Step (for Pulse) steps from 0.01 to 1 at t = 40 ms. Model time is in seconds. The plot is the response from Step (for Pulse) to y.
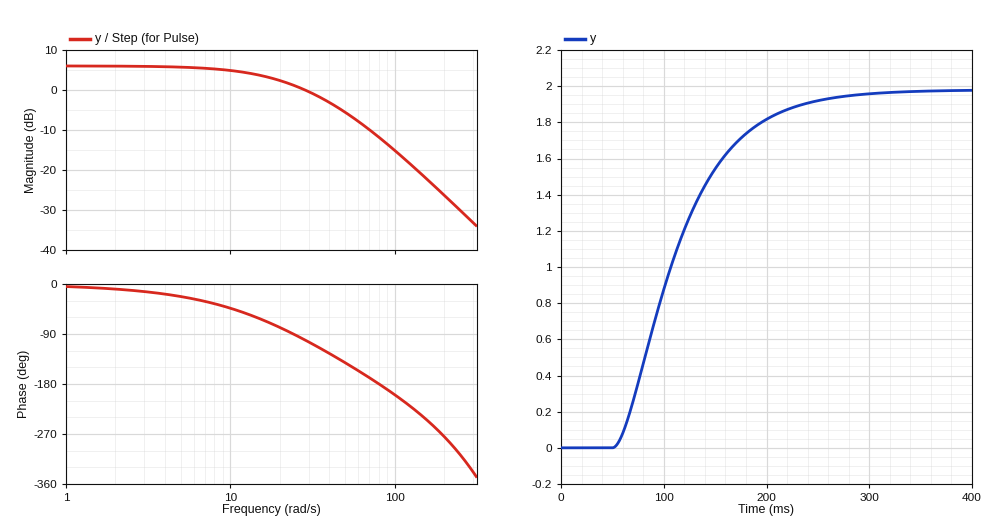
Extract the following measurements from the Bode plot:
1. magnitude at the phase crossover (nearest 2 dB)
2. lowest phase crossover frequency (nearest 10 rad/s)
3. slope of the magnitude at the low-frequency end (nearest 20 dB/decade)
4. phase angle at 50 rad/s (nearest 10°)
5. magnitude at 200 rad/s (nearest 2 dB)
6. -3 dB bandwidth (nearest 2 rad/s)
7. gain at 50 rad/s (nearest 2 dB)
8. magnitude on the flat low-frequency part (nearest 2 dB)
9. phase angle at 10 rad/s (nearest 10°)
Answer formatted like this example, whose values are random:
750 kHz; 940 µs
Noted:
-12 dB; 80 rad/s; 0 dB/decade; -140°; -26 dB; 18 rad/s; -6 dB; 6 dB; -40°
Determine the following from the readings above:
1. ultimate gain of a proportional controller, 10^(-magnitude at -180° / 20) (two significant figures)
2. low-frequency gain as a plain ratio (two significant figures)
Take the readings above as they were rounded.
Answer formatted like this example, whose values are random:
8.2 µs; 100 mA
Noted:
4.0; 2.0
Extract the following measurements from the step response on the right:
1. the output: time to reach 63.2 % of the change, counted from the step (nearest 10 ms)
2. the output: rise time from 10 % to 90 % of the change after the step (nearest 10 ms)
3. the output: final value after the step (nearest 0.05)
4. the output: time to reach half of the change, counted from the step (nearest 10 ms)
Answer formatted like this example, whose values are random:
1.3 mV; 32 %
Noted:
80 ms; 120 ms; 2.00; 70 ms
